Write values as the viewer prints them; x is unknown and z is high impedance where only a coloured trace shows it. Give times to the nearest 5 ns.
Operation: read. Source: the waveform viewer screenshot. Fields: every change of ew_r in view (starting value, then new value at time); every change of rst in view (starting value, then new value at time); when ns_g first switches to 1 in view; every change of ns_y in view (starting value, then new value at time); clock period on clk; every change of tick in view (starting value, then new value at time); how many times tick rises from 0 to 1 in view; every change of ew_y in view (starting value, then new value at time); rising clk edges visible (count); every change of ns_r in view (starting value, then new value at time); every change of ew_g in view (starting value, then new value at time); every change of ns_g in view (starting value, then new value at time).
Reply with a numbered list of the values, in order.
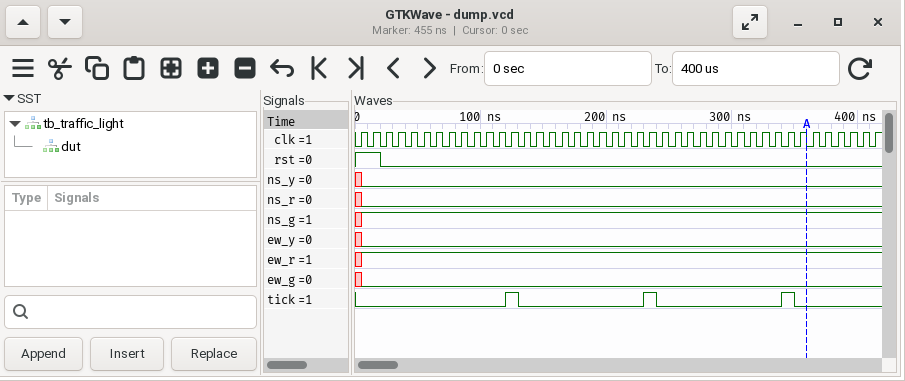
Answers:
1. x, 1 at 5 ns
2. 1, 0 at 20 ns
3. 5 ns
4. x, 0 at 5 ns
5. 10 ns
6. 0, 1 at 120 ns, 0 at 130 ns, 1 at 230 ns, 0 at 240 ns, 1 at 340 ns, 0 at 350 ns
7. 3
8. x, 0 at 5 ns
9. 42
10. x, 0 at 5 ns
11. x, 0 at 5 ns
12. x, 1 at 5 ns
